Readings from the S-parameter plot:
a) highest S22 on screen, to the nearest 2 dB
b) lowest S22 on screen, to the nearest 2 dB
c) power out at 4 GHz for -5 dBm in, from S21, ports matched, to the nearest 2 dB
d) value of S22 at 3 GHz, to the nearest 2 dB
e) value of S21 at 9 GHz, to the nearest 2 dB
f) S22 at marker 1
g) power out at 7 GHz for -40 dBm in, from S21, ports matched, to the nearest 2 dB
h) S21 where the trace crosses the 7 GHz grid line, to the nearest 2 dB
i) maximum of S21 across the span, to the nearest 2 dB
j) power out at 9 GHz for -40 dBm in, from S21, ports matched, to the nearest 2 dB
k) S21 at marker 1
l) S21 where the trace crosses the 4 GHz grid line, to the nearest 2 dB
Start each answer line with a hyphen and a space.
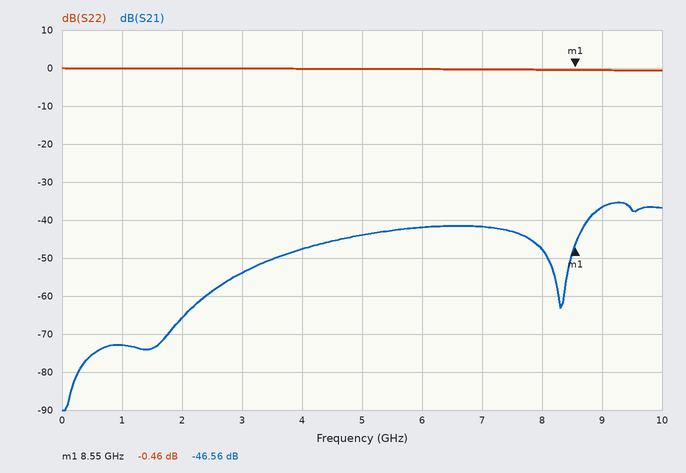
- 0 dB
- 0 dB
- -52 dBm
- 0 dB
- -36 dB
- -0.46 dB
- -82 dBm
- -42 dB
- -36 dB
- -76 dBm
- -46.56 dB
- -48 dB
